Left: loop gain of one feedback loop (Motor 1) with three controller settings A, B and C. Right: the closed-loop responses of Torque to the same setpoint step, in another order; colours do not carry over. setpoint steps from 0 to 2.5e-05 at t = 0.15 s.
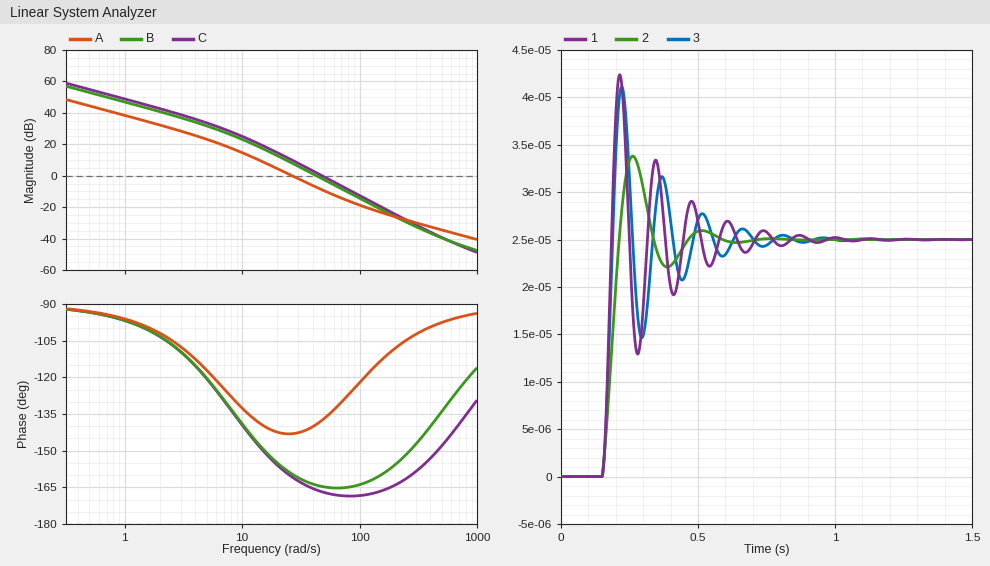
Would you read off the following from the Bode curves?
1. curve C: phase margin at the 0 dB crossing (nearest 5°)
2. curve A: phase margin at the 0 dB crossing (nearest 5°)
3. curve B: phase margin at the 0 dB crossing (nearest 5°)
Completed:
15°
35°
15°
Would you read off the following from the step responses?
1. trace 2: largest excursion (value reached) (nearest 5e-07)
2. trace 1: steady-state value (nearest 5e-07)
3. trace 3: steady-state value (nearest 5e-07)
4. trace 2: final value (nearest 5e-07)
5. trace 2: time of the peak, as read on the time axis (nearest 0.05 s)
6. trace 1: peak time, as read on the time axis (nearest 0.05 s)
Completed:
0.0000340
0.0000250
0.0000250
0.0000250
0.25 s
0.20 s
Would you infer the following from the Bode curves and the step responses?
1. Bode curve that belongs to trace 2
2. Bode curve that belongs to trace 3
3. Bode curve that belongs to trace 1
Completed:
A
B
C
